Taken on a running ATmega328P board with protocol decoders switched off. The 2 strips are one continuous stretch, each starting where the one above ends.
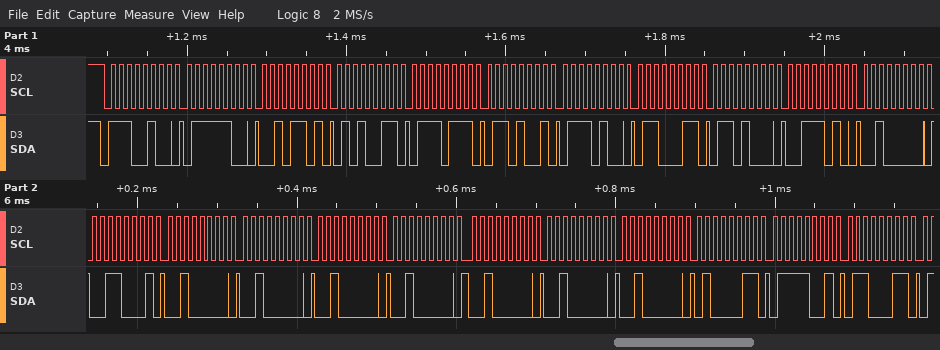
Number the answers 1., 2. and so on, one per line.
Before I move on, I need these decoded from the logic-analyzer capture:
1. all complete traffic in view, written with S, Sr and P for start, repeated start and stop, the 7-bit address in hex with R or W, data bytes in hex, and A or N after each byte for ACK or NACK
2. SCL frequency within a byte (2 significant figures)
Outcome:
1. S 72W A 7C A 2D A 53 A 77 A 69 A 74 A 63 A 68 A 3A A 20 A 31 A 20 A 20 A 20 A 20 A 20 A 20 A 20 A 43 A 79 A 63 A
2. 100 kHz
